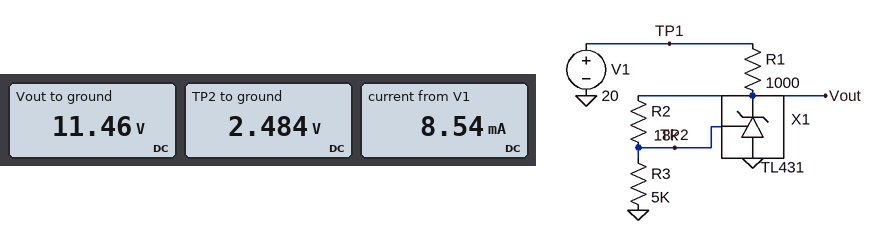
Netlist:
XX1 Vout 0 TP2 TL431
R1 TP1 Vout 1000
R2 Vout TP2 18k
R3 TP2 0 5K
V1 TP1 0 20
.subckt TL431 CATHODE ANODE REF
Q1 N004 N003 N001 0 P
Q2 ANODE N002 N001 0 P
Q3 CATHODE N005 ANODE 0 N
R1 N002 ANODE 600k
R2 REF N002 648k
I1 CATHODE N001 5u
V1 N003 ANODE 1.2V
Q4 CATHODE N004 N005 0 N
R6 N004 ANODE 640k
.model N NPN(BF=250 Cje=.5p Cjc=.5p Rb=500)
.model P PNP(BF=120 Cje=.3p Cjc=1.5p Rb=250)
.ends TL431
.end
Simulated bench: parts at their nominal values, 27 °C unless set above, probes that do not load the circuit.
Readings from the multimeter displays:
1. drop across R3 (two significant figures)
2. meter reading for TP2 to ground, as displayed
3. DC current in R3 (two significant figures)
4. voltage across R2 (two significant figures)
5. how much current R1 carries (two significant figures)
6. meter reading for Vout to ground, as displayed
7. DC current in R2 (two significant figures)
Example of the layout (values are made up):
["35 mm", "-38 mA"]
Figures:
["2.5 V", "2.484 V", "500 µA", "9.0 V", "8.5 mA", "11.46 V", "500 µA"]
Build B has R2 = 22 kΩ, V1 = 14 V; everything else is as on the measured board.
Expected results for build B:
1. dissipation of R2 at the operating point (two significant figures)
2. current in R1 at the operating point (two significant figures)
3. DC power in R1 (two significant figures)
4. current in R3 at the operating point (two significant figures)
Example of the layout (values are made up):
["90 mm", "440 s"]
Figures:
["5.4 mW", "660 µA", "440 µW", "490 µA"]
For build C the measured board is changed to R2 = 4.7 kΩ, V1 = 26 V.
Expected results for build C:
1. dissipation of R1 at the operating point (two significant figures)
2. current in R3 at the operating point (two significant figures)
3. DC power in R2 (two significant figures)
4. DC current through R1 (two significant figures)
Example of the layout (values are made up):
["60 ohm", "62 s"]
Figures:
["450 mW", "500 µA", "1.2 mW", "21 mA"]
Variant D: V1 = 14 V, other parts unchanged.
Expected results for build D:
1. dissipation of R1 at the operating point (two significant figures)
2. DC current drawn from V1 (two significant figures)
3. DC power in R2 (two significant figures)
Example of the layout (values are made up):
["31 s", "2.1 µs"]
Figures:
["6.7 mW", "2.6 mA", "4.4 mW"]
